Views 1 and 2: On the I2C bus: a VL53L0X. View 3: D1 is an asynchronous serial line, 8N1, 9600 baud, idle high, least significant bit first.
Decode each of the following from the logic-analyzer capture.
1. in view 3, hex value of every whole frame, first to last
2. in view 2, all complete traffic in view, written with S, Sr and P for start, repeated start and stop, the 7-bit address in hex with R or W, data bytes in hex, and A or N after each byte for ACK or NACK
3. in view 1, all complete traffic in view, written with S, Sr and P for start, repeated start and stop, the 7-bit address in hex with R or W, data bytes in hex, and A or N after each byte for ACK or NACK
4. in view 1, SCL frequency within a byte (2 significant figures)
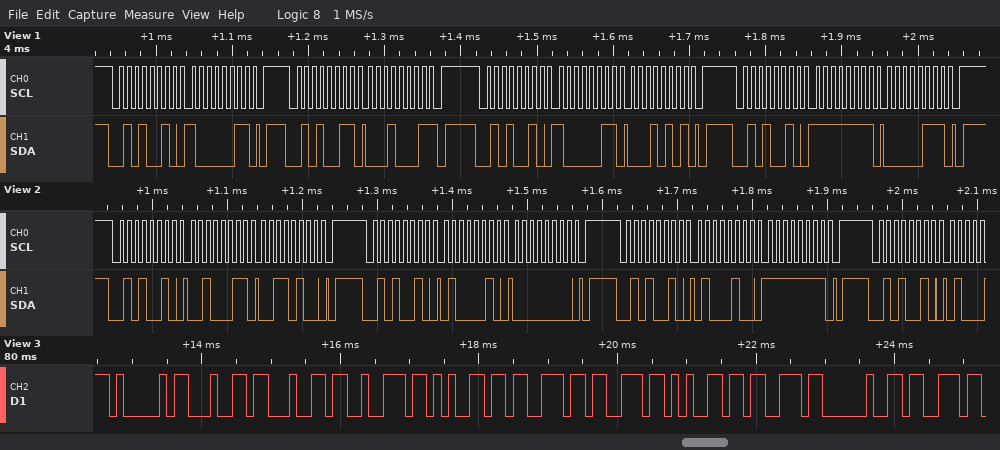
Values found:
41 64 64 72 65 73 73 65 73 20 73
S 29W A 23 A 34 A P S 29W A 42 A 00 A P S 29W A 44 A FF A P S 29W A
S 29W A 83 A P S 29R A 11 N P S 29W A 83 A 15 A P S 29W A FF A 07 A P
100 kHz
